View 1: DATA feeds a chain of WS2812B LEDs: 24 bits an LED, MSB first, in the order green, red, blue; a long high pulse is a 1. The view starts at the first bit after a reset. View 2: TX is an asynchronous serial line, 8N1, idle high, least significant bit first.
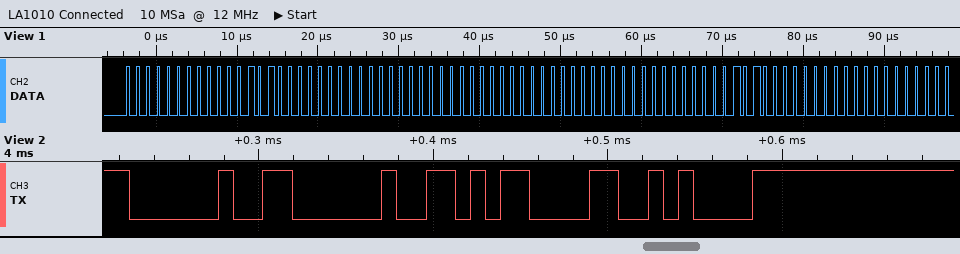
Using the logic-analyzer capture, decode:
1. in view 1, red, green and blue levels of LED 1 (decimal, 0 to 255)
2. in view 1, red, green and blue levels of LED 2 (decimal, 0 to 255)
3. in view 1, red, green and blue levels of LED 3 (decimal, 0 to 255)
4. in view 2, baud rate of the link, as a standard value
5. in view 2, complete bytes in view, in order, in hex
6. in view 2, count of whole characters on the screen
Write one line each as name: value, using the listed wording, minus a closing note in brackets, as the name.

in view 1, red, green and blue levels of LED 1: 10, 0, 0
in view 1, red, green and blue levels of LED 2: 0, 0, 0
in view 1, red, green and blue levels of LED 3: 10, 0, 0
in view 2, baud rate of the link, as a standard value: 115200 baud
in view 2, complete bytes in view, in order, in hex: 0x20 0x20 0x0D 0x0A
in view 2, count of whole characters on the screen: 4
